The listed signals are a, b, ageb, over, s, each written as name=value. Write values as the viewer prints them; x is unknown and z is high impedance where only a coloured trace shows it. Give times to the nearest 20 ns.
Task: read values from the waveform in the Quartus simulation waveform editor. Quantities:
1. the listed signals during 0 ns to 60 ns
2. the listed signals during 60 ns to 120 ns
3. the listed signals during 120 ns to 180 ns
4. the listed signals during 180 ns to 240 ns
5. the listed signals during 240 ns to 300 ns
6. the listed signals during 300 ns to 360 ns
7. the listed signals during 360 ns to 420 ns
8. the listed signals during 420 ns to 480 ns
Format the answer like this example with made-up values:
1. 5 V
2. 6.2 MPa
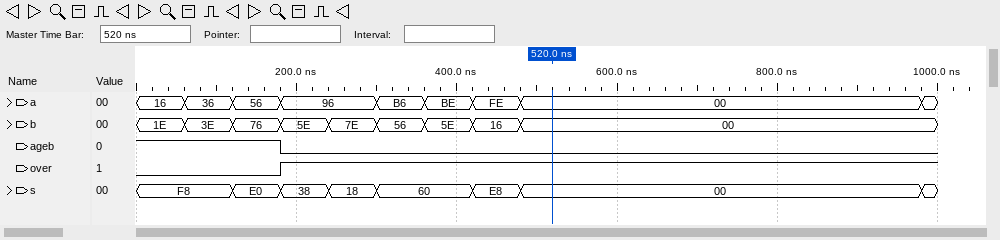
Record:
1. a=16, b=1E, ageb=1, over=0, s=F8
2. a=36, b=3E, ageb=1, over=0, s=F8
3. a=56, b=76, ageb=1, over=0, s=E0
4. a=96, b=5E, ageb=0, over=1, s=38
5. a=96, b=7E, ageb=0, over=1, s=18
6. a=B6, b=56, ageb=0, over=1, s=60
7. a=BE, b=5E, ageb=0, over=1, s=60
8. a=FE, b=16, ageb=0, over=1, s=E8
